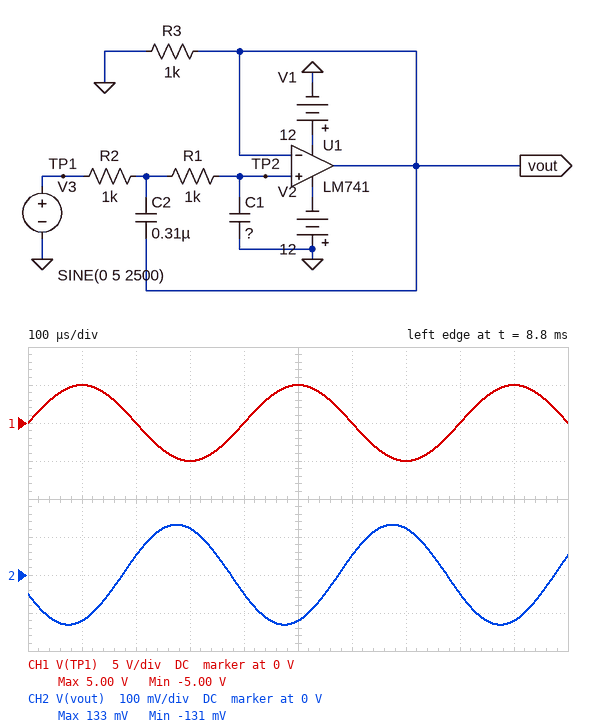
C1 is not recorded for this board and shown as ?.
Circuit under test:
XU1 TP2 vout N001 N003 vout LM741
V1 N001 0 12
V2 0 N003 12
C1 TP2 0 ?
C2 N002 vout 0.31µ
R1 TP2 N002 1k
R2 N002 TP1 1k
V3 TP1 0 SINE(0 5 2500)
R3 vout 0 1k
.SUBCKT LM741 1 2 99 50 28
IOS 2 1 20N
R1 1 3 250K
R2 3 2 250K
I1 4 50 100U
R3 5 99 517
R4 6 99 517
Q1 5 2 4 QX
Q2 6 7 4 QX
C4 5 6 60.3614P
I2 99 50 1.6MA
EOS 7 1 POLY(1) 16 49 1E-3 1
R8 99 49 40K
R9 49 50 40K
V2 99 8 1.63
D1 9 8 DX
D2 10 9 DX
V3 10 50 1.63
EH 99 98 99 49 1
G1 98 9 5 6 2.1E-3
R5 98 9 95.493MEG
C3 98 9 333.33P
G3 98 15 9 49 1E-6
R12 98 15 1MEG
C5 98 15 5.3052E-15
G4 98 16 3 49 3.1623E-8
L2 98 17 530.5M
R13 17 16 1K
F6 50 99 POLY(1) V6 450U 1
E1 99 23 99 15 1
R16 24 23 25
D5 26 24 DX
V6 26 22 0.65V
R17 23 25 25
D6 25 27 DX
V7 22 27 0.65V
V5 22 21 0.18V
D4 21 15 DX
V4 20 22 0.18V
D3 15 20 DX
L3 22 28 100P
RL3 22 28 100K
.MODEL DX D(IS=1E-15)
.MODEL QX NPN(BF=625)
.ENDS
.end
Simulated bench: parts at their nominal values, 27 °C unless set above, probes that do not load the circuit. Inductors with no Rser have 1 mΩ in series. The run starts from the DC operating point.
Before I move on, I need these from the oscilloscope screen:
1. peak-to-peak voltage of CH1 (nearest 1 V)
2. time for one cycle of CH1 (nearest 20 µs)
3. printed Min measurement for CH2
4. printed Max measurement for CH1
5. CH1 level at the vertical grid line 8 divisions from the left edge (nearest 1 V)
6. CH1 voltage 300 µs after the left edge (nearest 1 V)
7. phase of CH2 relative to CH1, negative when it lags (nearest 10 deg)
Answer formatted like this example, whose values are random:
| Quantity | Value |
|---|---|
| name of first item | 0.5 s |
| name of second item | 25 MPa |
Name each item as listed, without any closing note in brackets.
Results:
| Quantity | Value |
|---|---|
| peak-to-peak voltage of CH1 | 10 V |
| time for one cycle of CH1 | 400 µs |
| printed Min measurement for CH2 | -131 mV |
| printed Max measurement for CH1 | 5.00 V |
| CH1 level at the vertical grid line 8 divisions from the left edge | 0 V |
| CH1 voltage 300 µs after the left edge | -5 V |
| phase of CH2 relative to CH1, negative when it lags | -160 deg |
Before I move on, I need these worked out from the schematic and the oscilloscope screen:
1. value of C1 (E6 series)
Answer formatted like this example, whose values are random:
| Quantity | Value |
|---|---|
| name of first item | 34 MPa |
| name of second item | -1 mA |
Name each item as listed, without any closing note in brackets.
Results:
| Quantity | Value |
|---|---|
| value of C1 | 470 nF |
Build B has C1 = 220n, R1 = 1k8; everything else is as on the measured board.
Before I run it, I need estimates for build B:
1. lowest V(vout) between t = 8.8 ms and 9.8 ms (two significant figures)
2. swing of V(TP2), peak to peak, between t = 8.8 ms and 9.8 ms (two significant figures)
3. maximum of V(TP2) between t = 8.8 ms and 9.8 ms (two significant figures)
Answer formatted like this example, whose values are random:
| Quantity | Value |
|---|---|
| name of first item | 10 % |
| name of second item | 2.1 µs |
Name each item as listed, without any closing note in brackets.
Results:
| Quantity | Value |
|---|---|
| lowest V(vout) between t = 8.8 ms and 9.8 ms | -160 mV |
| swing of V(TP2), peak to peak, between t = 8.8 ms and 9.8 ms | 320 mV |
| maximum of V(TP2) between t = 8.8 ms and 9.8 ms | 160 mV |
